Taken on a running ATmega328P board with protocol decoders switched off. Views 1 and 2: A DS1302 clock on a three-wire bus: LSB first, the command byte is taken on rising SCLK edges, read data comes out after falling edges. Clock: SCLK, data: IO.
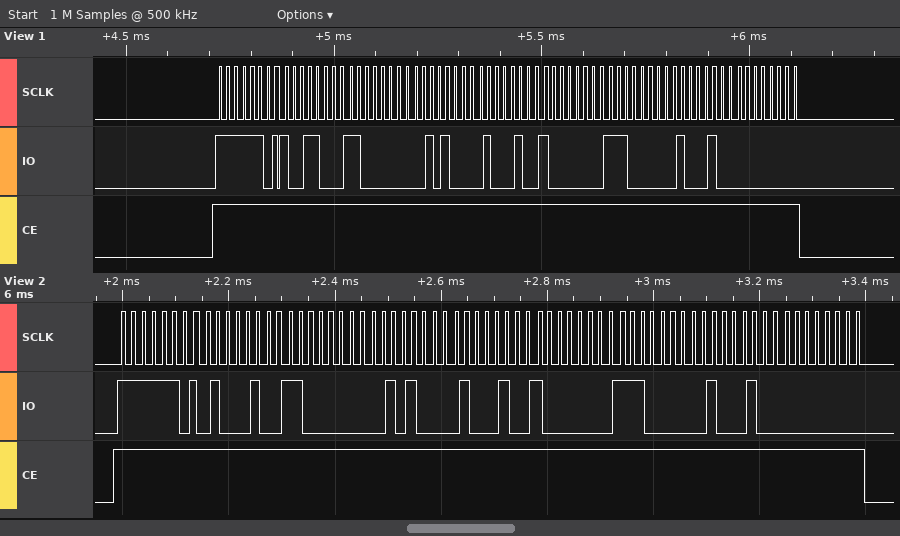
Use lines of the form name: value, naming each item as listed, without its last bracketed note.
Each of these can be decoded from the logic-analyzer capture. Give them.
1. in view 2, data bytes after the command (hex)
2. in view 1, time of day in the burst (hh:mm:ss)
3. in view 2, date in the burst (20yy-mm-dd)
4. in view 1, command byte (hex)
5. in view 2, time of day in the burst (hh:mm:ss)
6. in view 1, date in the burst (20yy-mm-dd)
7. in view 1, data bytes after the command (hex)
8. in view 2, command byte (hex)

in view 2, data bytes after the command: 22 03 14 22 01 07 22 00
in view 1, time of day in the burst: 14:03:19
in view 2, date in the burst: 2022-01-22
in view 1, command byte: 0xBF
in view 2, time of day in the burst: 14:03:22
in view 1, date in the burst: 2022-01-22
in view 1, data bytes after the command: 19 03 14 22 01 07 22 00
in view 2, command byte: 0xBF
